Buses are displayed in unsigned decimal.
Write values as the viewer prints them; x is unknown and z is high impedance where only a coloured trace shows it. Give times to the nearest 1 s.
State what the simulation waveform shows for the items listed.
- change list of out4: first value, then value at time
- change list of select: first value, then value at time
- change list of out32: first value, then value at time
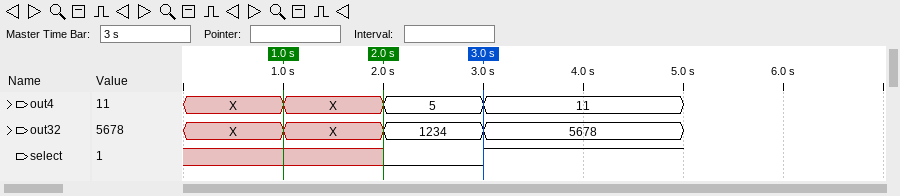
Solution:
X, X at 1 s, 5 at 2 s, 11 at 3 s
x, 0 at 2 s, 1 at 3 s
X, X at 1 s, 1234 at 2 s, 5678 at 3 s
